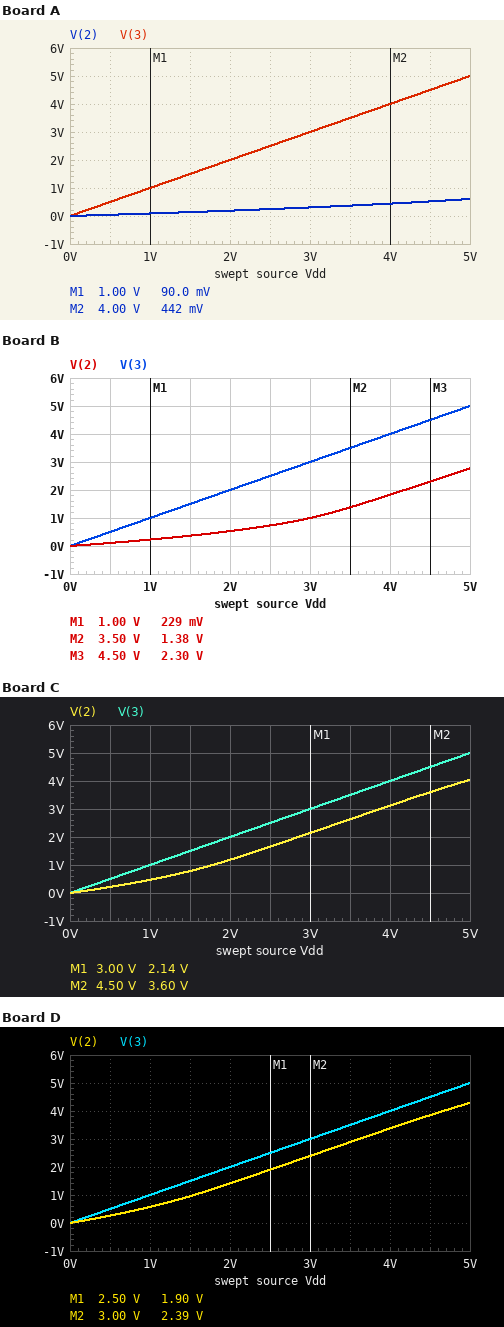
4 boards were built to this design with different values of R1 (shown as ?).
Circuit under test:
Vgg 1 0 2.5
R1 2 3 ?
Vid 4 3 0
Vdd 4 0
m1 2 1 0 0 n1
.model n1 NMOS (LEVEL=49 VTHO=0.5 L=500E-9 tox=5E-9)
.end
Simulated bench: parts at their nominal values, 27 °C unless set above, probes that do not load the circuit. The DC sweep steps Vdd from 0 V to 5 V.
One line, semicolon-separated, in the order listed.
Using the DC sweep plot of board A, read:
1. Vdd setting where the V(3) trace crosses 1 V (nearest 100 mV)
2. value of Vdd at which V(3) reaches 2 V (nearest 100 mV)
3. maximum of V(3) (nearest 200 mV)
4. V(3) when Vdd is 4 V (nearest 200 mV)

1.0 V; 2.0 V; 5.0 V; 4.0 V
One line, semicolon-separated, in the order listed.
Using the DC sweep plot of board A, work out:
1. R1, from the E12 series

3.3 kΩ
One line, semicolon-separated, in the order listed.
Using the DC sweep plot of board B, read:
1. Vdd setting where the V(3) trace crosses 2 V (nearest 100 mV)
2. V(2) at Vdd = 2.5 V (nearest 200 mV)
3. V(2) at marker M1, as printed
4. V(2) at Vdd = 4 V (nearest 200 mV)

2.0 V; 800 mV; 229 mV; 1.8 V
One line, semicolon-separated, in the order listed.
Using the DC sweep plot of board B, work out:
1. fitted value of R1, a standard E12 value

1.2 kΩ
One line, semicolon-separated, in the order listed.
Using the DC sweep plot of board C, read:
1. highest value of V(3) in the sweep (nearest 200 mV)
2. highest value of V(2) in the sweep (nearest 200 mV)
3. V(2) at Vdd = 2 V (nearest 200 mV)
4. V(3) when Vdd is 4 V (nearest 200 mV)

5.0 V; 4.0 V; 1.2 V; 4.0 V
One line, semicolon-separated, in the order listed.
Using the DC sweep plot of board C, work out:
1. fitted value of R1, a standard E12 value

470 Ω
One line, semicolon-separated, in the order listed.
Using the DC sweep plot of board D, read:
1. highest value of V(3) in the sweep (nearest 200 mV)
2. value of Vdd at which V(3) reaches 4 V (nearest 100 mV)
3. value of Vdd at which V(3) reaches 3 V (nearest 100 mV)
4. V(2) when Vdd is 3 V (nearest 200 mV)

5.0 V; 4.0 V; 3.0 V; 2.4 V
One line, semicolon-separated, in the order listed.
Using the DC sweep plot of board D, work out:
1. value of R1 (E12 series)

330 Ω
